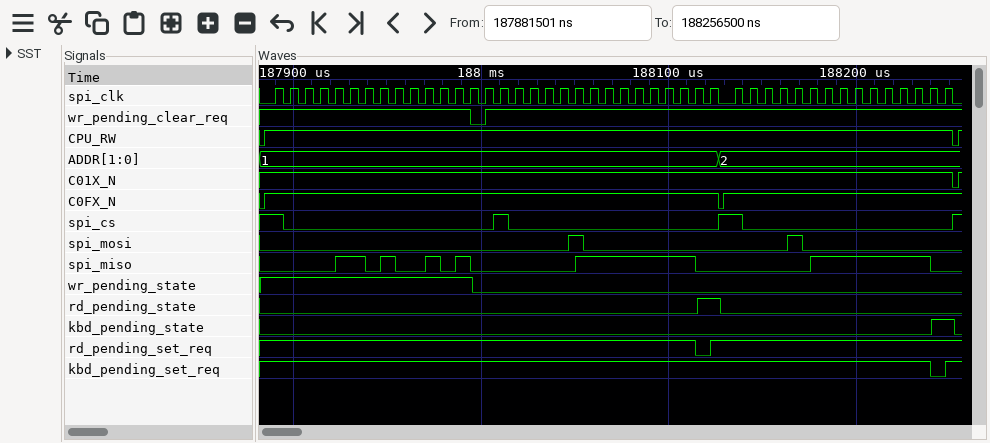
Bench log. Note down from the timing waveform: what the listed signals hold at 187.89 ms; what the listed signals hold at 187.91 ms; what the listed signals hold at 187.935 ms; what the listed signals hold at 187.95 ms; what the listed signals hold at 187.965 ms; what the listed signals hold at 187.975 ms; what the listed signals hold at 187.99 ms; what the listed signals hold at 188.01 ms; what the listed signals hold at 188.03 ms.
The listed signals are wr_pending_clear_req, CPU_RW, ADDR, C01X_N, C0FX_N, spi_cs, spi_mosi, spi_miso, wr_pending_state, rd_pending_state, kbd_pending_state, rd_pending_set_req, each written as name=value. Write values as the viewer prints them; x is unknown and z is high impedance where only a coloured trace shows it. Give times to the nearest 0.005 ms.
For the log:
wr_pending_clear_req=1, CPU_RW=1, ADDR=1, C01X_N=1, C0FX_N=1, spi_cs=1, spi_mosi=0, spi_miso=0, wr_pending_state=1, rd_pending_state=0, kbd_pending_state=0, rd_pending_set_req=1
wr_pending_clear_req=1, CPU_RW=1, ADDR=1, C01X_N=1, C0FX_N=1, spi_cs=0, spi_mosi=0, spi_miso=0, wr_pending_state=1, rd_pending_state=0, kbd_pending_state=0, rd_pending_set_req=1
wr_pending_clear_req=1, CPU_RW=1, ADDR=1, C01X_N=1, C0FX_N=1, spi_cs=0, spi_mosi=0, spi_miso=1, wr_pending_state=1, rd_pending_state=0, kbd_pending_state=0, rd_pending_set_req=1
wr_pending_clear_req=1, CPU_RW=1, ADDR=1, C01X_N=1, C0FX_N=1, spi_cs=0, spi_mosi=0, spi_miso=1, wr_pending_state=1, rd_pending_state=0, kbd_pending_state=0, rd_pending_set_req=1
wr_pending_clear_req=1, CPU_RW=1, ADDR=1, C01X_N=1, C0FX_N=1, spi_cs=0, spi_mosi=0, spi_miso=0, wr_pending_state=1, rd_pending_state=0, kbd_pending_state=0, rd_pending_set_req=1
wr_pending_clear_req=1, CPU_RW=1, ADDR=1, C01X_N=1, C0FX_N=1, spi_cs=0, spi_mosi=0, spi_miso=1, wr_pending_state=1, rd_pending_state=0, kbd_pending_state=0, rd_pending_set_req=1
wr_pending_clear_req=1, CPU_RW=1, ADDR=1, C01X_N=1, C0FX_N=1, spi_cs=0, spi_mosi=0, spi_miso=1, wr_pending_state=1, rd_pending_state=0, kbd_pending_state=0, rd_pending_set_req=1
wr_pending_clear_req=1, CPU_RW=1, ADDR=1, C01X_N=1, C0FX_N=1, spi_cs=1, spi_mosi=0, spi_miso=0, wr_pending_state=0, rd_pending_state=0, kbd_pending_state=0, rd_pending_set_req=1
wr_pending_clear_req=1, CPU_RW=1, ADDR=1, C01X_N=1, C0FX_N=1, spi_cs=0, spi_mosi=0, spi_miso=0, wr_pending_state=0, rd_pending_state=0, kbd_pending_state=0, rd_pending_set_req=1
